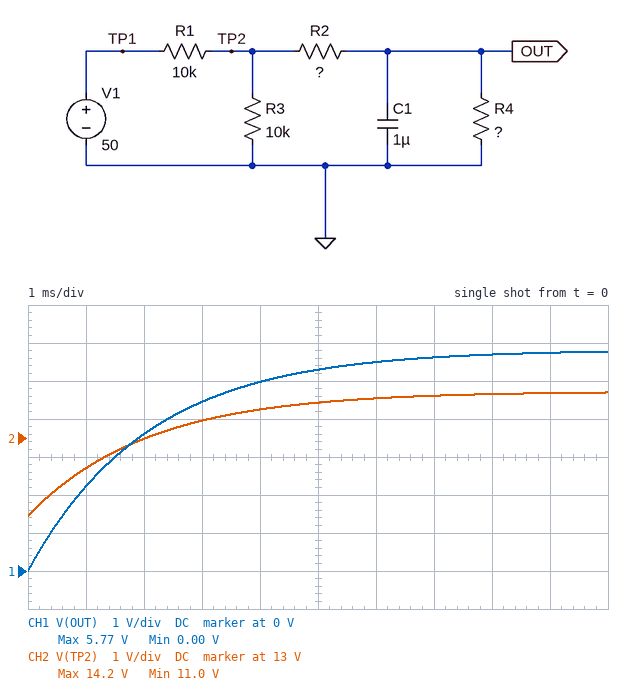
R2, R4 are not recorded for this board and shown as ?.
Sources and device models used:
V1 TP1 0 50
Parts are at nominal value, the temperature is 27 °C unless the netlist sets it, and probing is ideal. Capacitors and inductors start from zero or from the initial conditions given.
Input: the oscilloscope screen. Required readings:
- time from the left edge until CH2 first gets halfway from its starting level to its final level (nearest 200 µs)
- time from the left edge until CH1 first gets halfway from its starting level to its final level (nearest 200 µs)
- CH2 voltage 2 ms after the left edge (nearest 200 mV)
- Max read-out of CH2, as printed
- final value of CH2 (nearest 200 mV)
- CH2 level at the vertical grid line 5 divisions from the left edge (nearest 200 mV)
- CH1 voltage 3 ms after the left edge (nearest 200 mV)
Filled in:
1.4 ms
1.4 ms
13.0 V
14.2 V
14.2 V
14.0 V
4.4 V
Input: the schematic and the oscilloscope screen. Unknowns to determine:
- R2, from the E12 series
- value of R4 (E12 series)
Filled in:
3.9 kΩ
2.7 kΩ
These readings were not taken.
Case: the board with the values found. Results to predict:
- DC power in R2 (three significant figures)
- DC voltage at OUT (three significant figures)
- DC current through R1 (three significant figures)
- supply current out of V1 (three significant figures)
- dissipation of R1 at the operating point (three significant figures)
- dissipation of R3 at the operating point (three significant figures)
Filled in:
18.1 mW
5.82 V
3.58 mA
3.58 mA
128 mW
20.2 mW
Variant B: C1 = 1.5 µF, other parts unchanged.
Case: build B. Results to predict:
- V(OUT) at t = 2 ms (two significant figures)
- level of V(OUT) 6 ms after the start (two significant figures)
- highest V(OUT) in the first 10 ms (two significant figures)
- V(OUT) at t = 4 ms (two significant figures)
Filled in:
2.8 V
5.0 V
5.6 V
4.2 V
